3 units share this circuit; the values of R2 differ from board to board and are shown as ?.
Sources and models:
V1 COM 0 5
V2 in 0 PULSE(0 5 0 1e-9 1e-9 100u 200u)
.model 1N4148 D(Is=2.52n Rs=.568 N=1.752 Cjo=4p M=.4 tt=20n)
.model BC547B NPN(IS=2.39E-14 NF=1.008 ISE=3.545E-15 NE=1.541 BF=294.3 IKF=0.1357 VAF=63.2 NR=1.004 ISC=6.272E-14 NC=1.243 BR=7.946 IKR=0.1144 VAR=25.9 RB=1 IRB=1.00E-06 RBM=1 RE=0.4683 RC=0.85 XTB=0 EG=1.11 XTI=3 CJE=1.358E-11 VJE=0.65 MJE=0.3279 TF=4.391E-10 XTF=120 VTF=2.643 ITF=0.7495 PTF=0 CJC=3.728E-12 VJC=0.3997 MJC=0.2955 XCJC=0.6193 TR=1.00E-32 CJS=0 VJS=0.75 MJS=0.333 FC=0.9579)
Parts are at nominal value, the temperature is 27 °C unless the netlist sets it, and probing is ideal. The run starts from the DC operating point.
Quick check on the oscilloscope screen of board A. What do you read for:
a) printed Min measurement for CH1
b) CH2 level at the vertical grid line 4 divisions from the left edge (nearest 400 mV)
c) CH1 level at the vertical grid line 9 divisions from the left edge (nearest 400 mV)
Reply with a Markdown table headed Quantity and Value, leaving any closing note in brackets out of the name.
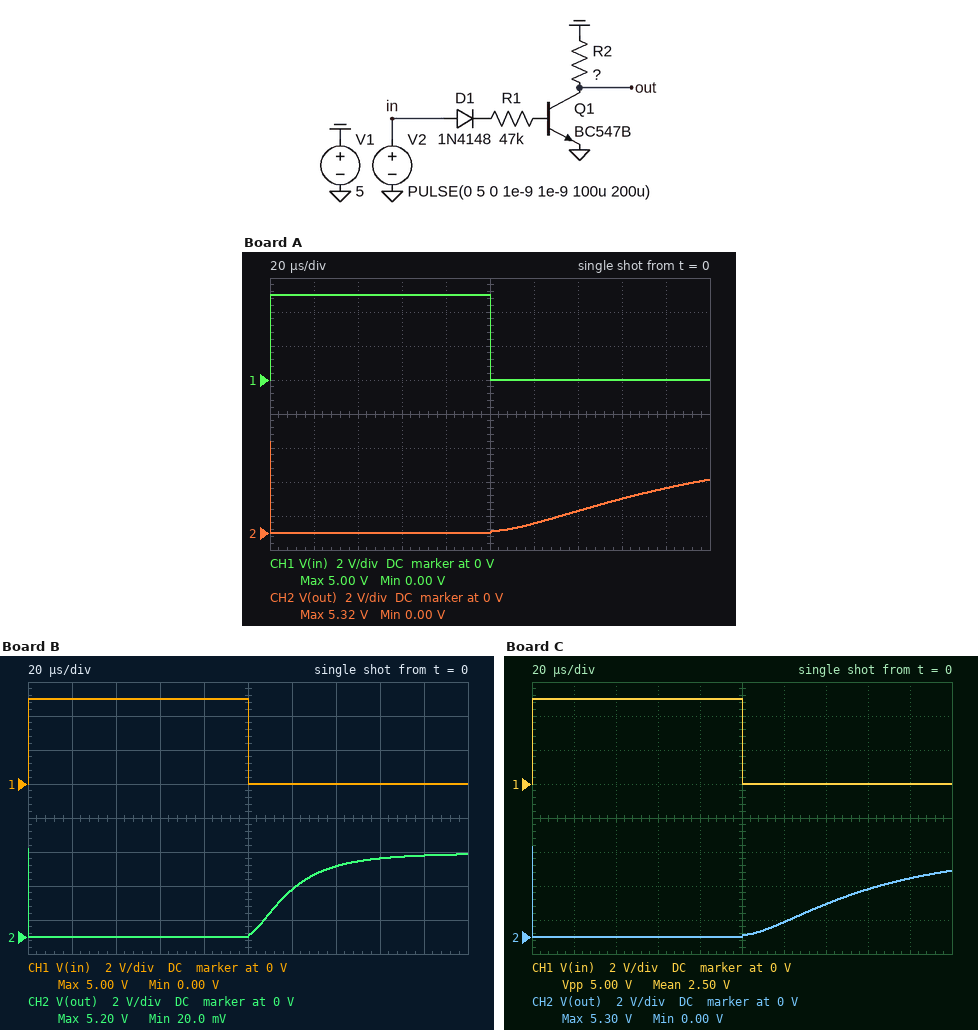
| Quantity | Value |
|---|---|
| printed Min measurement for CH1 | 0.00 V |
| CH2 level at the vertical grid line 4 divisions from the left edge | 0 V |
| CH1 level at the vertical grid line 9 divisions from the left edge | 0 V |
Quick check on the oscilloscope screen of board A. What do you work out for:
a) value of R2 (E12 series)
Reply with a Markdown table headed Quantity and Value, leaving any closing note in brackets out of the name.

| Quantity | Value |
|---|---|
| value of R2 | 120 kΩ |
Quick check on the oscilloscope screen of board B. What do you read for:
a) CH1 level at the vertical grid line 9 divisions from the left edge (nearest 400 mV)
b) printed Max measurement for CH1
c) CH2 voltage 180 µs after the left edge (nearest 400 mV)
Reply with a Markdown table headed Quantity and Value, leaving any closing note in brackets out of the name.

| Quantity | Value |
|---|---|
| CH1 level at the vertical grid line 9 divisions from the left edge | 0 V |
| printed Max measurement for CH1 | 5.00 V |
| CH2 voltage 180 µs after the left edge | 4.8 V |
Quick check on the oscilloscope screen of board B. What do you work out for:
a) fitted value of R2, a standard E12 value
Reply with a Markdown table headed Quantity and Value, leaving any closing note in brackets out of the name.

| Quantity | Value |
|---|---|
| fitted value of R2, a standard E12 value | 27 kΩ |
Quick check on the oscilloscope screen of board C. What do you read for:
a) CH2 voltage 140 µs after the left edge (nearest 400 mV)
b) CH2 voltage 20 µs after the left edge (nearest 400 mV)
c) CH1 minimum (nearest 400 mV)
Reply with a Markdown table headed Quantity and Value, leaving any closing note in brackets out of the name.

| Quantity | Value |
|---|---|
| CH2 voltage 140 µs after the left edge | 2.0 V |
| CH2 voltage 20 µs after the left edge | 0 V |
| CH1 minimum | 0 V |
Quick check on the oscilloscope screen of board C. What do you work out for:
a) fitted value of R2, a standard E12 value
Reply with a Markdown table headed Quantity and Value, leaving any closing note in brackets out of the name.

| Quantity | Value |
|---|---|
| fitted value of R2, a standard E12 value | 82 kΩ |
